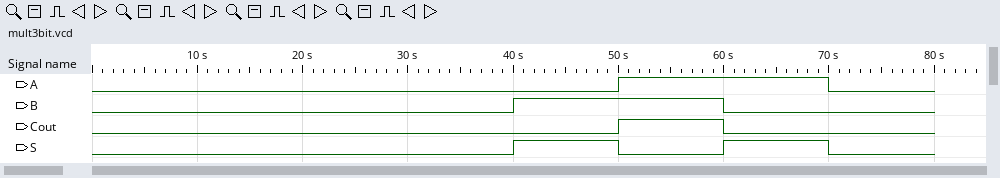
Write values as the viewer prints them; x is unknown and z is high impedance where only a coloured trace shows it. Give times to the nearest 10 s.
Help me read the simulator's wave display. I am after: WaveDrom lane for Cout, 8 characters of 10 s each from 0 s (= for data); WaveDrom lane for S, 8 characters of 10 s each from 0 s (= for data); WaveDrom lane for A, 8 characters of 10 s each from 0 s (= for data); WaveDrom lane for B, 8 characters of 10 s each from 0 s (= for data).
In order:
{name: 'Cout', wave: '0....10.'}
{name: 'S', wave: '0...1010'}
{name: 'A', wave: '0....1.0'}
{name: 'B', wave: '0...1.0.'}
